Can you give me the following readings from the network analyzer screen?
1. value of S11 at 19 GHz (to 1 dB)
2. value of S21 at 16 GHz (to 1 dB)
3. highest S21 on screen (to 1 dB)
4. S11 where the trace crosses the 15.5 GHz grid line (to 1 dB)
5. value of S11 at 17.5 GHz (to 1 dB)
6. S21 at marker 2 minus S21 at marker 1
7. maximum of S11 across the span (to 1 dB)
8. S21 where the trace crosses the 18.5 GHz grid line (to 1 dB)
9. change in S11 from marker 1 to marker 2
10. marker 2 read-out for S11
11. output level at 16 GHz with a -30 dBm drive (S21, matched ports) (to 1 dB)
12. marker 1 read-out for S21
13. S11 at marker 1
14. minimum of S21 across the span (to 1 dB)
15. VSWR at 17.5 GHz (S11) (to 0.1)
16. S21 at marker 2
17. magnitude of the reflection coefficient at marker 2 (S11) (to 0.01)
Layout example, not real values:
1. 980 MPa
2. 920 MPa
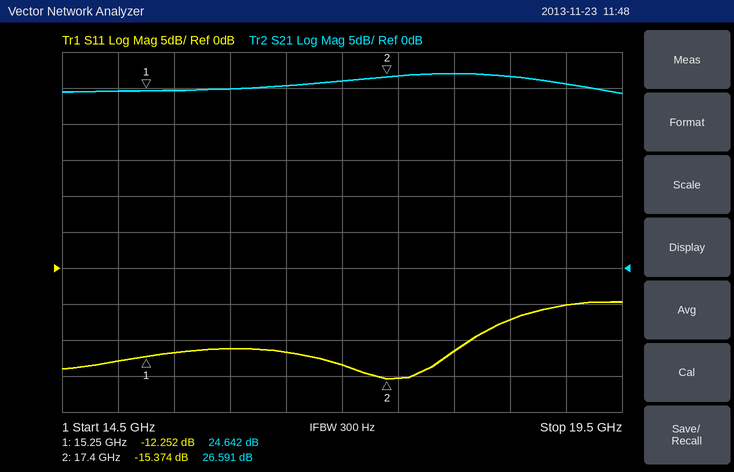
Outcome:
1. -5 dB
2. 25 dB
3. 27 dB
4. -12 dB
5. -15 dB
6. 1.949 dB
7. -5 dB
8. 27 dB
9. -3.122 dB
10. -15.374 dB
11. -5 dBm
12. 24.642 dB
13. -12.252 dB
14. 24 dB
15. 1.4
16. 26.591 dB
17. 0.17
